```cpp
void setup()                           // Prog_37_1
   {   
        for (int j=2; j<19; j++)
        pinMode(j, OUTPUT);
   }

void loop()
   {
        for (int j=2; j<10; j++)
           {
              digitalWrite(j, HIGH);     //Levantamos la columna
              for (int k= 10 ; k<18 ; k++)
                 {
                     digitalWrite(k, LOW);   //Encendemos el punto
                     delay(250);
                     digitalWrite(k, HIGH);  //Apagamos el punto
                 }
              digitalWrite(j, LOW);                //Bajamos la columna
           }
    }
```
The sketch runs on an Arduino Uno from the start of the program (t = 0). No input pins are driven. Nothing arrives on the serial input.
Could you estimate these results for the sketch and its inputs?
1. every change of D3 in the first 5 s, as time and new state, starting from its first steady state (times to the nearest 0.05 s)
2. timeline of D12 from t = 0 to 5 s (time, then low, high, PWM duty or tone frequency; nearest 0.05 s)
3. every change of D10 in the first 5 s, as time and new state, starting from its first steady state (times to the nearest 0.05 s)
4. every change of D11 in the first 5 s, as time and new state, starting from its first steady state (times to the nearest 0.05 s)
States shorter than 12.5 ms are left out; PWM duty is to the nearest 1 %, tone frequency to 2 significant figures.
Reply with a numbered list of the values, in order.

1. 0 s low; 2 s high; 4 s low
2. 0 s low; 0.75 s high; 2.5 s low; 2.75 s high; 4.5 s low; 4.75 s high
3. 0 s low; 0.25 s high; 2 s low; 2.25 s high; 4 s low; 4.25 s high
4. 0 s low; 0.5 s high; 2.25 s low; 2.5 s high; 4.25 s low; 4.5 s high
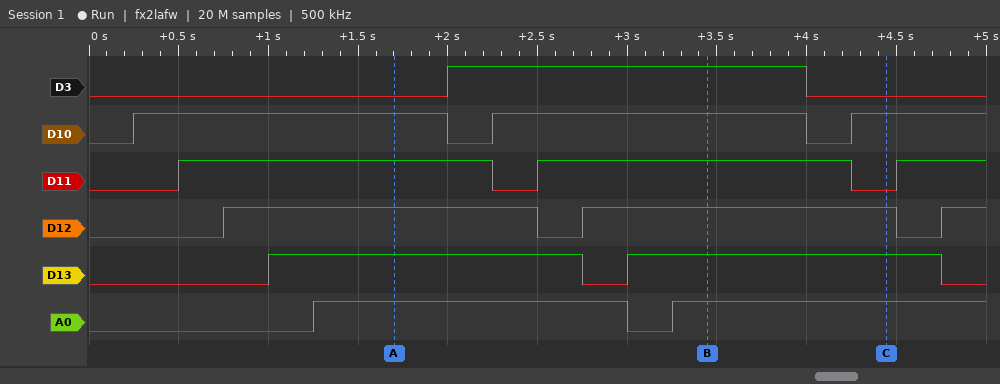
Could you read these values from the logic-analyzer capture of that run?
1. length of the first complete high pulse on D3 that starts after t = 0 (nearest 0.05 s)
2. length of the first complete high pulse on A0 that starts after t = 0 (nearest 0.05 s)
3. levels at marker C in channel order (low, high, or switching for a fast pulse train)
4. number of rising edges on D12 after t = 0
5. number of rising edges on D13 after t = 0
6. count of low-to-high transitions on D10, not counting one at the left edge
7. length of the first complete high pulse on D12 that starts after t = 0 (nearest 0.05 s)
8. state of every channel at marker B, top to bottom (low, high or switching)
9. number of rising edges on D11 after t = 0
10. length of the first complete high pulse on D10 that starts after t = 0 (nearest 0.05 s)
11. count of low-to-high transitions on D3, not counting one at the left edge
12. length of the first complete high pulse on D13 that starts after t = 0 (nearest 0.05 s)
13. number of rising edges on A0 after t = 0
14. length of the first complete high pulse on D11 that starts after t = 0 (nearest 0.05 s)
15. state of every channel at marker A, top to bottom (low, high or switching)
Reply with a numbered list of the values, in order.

1. 2.00 s
2. 1.75 s
3. D3 low, D10 high, D11 low, D12 high, D13 high, A0 high
4. 3
5. 2
6. 3
7. 1.75 s
8. D3 high, D10 high, D11 high, D12 high, D13 high, A0 high
9. 3
10. 1.75 s
11. 1
12. 1.75 s
13. 2
14. 1.75 s
15. D3 low, D10 high, D11 high, D12 high, D13 high, A0 high
